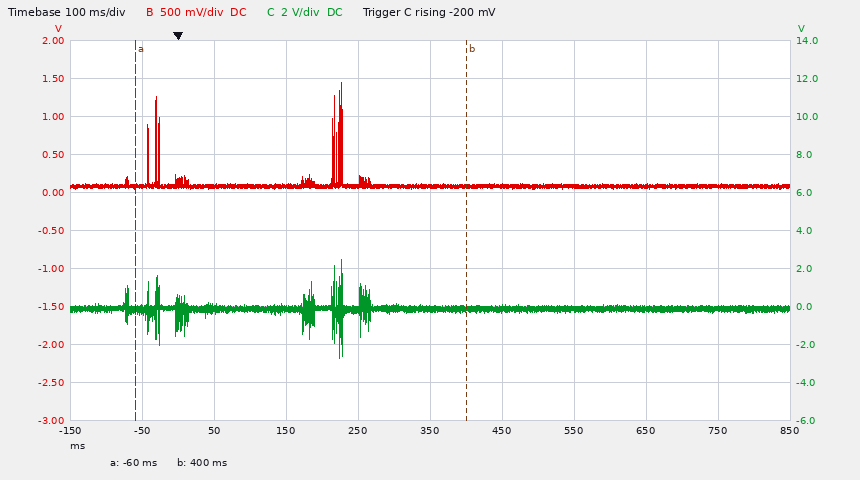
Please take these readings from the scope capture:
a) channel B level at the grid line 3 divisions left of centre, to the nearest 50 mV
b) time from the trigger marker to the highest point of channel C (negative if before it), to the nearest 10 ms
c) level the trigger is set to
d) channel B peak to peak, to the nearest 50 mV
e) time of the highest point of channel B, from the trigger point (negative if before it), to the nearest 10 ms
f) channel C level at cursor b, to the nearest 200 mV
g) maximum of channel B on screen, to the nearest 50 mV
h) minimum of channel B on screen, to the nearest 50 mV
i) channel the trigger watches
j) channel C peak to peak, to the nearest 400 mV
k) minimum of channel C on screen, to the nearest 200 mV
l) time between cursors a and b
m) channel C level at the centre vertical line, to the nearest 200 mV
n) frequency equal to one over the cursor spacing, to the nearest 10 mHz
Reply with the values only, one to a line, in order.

100 mV
+230 ms
-200 mV
1.40 V
+230 ms
-200 mV
1.45 V
50 mV
channel C
5.2 V
-2.8 V
460 ms
-200 mV
2.17 Hz
